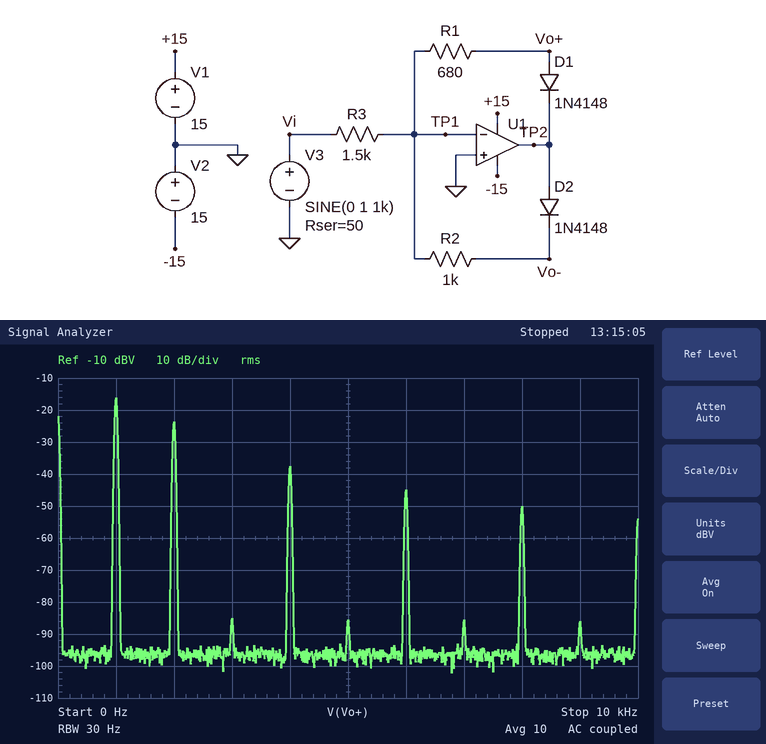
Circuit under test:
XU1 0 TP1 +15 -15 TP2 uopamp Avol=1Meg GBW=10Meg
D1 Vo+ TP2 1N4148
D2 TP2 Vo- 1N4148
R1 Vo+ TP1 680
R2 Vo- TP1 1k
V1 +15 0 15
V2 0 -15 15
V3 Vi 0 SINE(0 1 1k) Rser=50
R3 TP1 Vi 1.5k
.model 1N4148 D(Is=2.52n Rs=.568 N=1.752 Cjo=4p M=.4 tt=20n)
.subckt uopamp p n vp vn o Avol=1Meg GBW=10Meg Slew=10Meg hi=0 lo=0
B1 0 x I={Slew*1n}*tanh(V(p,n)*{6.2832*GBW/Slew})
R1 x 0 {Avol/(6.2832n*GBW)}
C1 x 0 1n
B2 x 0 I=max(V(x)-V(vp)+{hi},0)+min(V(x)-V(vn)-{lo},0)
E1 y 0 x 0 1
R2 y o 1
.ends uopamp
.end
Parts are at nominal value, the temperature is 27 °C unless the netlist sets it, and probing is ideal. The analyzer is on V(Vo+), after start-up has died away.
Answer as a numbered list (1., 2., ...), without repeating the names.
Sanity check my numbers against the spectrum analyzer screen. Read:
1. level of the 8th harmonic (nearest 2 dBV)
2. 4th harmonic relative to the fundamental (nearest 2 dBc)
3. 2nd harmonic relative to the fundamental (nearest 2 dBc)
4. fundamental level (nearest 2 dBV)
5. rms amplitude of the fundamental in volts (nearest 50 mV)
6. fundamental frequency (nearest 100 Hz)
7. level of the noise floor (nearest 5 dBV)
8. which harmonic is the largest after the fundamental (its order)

1. -50 dBV
2. -22 dBc
3. -8 dBc
4. -16 dBV
5. 150 mV
6. 1.0 kHz
7. -95 dBV
8. 2
